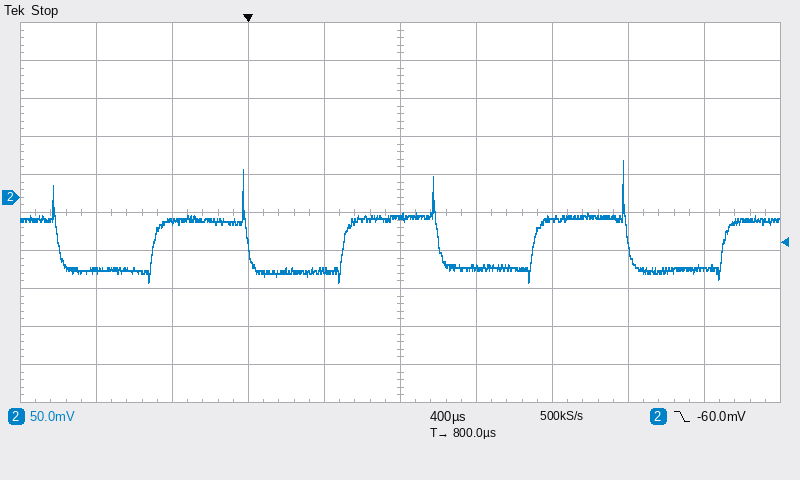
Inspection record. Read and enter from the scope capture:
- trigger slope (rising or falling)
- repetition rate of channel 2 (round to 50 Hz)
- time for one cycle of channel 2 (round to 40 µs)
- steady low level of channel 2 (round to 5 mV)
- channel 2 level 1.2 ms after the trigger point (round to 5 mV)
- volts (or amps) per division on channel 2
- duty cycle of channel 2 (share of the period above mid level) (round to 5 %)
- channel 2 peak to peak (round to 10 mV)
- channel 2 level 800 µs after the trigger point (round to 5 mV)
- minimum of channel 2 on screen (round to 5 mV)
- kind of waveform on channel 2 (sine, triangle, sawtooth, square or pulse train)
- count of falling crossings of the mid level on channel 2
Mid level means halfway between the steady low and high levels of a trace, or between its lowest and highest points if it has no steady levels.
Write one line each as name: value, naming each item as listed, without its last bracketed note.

trigger slope: falling
repetition rate of channel 2: 1.00 kHz
time for one cycle of channel 2: 1.00 ms
steady low level of channel 2: -95 mV
channel 2 level 1.2 ms after the trigger point: -90 mV
volts (or amps) per division on channel 2: 50 mV
duty cycle of channel 2 (share of the period above mid level): 50 %
channel 2 peak to peak: 160 mV
channel 2 level 800 µs after the trigger point: -25 mV
minimum of channel 2 on screen: -110 mV
kind of waveform on channel 2: square
count of falling crossings of the mid level on channel 2: 4
